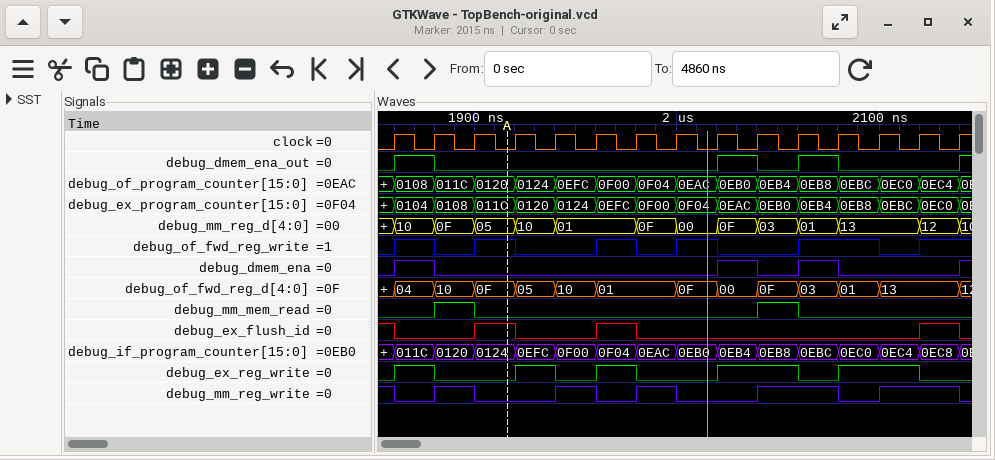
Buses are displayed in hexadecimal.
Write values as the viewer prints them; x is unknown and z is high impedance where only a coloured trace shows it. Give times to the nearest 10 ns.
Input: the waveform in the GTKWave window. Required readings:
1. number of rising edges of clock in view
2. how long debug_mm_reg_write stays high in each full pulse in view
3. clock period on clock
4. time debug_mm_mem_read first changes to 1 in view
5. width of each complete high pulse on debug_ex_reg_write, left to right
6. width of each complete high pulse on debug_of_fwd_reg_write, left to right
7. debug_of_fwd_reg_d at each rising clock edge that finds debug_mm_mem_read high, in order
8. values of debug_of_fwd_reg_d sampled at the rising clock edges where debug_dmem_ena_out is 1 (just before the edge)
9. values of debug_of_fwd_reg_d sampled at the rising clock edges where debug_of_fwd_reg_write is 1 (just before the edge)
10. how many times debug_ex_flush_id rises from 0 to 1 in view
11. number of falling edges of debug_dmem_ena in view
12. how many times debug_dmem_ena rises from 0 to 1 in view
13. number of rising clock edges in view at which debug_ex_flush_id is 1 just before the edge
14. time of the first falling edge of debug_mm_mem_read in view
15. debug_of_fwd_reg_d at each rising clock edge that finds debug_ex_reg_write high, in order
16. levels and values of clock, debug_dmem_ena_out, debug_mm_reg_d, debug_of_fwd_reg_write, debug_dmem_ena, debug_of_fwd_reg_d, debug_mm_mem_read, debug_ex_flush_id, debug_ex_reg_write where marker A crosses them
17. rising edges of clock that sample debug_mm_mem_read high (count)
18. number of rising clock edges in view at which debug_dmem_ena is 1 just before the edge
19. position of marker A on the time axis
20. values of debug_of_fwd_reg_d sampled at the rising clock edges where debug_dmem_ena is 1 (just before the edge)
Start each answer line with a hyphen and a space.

- 15
- 20 ns, 20 ns, 20 ns, 40 ns, 40 ns
- 20 ns
- 1880 ns
- 20 ns, 20 ns, 20 ns, 40 ns, 40 ns
- 20 ns, 20 ns, 20 ns, 20 ns, 40 ns
- 10, 0F
- 04, 00, 03
- 04, 0F, 01, 0F, 03, 01, 13
- 3
- 3
- 4
- 4
- 1900 ns
- 04, 05, 01, 00, 0F, 01, 13
- clock=0, debug_dmem_ena_out=0, debug_mm_reg_d=05, debug_of_fwd_reg_write=1, debug_dmem_ena=0, debug_of_fwd_reg_d=0F, debug_mm_mem_read=0, debug_ex_flush_id=1, debug_ex_reg_write=0
- 2
- 3
- 1920 ns
- 04, 00, 03
